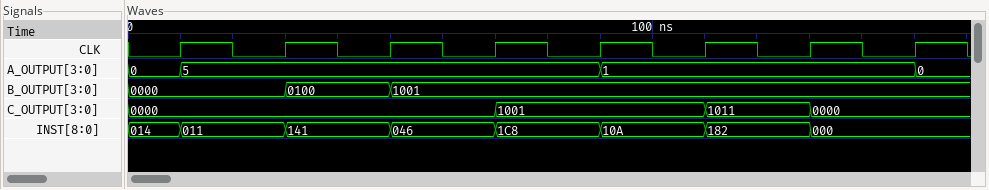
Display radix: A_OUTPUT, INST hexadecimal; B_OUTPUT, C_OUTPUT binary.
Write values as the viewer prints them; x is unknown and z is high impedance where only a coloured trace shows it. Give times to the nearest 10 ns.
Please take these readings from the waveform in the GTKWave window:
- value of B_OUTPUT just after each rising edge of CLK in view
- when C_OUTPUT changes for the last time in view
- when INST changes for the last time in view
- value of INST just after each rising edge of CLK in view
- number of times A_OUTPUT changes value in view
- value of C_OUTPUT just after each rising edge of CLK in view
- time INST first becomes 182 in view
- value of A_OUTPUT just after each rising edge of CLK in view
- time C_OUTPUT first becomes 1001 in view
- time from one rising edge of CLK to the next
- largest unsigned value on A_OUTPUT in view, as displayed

0000, 0100, 1001, 1001, 1001, 1001, 1001, 1001
130 ns
130 ns
011, 141, 046, 1C8, 10A, 182, 000, 000
3
0000, 0000, 0000, 1001, 1001, 1011, 0000, 0000
110 ns
5, 5, 5, 5, 1, 1, 1, 0
70 ns
20 ns
5
